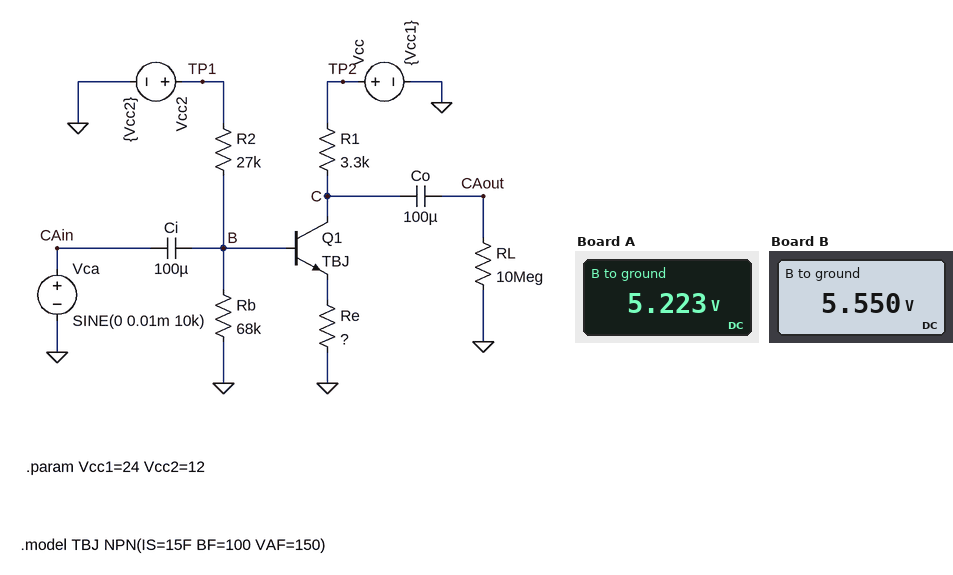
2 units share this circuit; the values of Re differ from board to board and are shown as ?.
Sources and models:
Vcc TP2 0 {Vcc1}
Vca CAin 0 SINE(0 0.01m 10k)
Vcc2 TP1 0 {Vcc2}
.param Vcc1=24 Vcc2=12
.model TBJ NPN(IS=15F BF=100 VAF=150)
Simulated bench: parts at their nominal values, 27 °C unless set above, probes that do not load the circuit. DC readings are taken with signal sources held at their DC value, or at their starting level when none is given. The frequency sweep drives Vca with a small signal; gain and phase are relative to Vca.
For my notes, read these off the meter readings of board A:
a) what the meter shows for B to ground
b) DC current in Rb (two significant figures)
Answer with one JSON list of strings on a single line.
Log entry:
["5.223 V", "77 µA"]
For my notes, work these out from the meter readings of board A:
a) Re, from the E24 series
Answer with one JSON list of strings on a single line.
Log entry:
["750 Ω"]
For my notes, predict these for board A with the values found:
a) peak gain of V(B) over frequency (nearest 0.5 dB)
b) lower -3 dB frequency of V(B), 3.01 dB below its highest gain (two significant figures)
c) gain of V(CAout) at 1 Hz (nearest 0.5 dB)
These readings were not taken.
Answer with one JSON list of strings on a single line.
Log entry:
["0 dB", "2.5 Hz", "-12.0 dB"]
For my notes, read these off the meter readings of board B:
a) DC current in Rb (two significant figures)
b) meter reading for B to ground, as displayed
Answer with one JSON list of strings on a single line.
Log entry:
["82 µA", "5.550 V"]
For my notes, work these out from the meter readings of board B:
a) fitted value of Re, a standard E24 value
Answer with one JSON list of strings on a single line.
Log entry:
["820 Ω"]
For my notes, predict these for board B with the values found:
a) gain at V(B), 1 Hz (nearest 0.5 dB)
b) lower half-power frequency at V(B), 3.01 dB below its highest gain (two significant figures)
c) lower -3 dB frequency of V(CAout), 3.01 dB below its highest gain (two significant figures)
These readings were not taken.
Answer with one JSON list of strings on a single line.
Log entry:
["-8.0 dB", "2.3 Hz", "2.3 Hz"]
